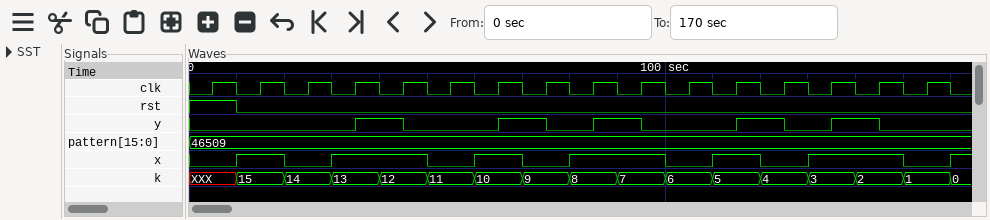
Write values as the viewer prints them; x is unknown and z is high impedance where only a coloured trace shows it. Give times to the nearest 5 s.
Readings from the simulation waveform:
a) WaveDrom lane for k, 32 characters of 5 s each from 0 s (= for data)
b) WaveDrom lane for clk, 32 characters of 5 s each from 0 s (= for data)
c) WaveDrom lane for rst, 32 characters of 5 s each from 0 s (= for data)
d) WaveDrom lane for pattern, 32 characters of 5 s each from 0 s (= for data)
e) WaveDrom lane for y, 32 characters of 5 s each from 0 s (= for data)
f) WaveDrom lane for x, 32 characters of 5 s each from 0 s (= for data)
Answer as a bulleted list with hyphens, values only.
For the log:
- {name: 'k', wave: 'x.=.=.=.=.=.=.=.=.=.=.=.=.=.=.=.', data: '15 14 13 12 11 10 9 8 7 6 5 4 3 2 1'}
- {name: 'clk', wave: '01010101010101010101010101010101'}
- {name: 'rst', wave: '1.0.............................'}
- {name: 'pattern', wave: '=...............................', data: '46509'}
- {name: 'y', wave: '0......1.0...1.0.1.0...1.0.1.0..'}
- {name: 'x', wave: '0.1.0.1...0.1.0.1...0.1.0.1...0.'}
